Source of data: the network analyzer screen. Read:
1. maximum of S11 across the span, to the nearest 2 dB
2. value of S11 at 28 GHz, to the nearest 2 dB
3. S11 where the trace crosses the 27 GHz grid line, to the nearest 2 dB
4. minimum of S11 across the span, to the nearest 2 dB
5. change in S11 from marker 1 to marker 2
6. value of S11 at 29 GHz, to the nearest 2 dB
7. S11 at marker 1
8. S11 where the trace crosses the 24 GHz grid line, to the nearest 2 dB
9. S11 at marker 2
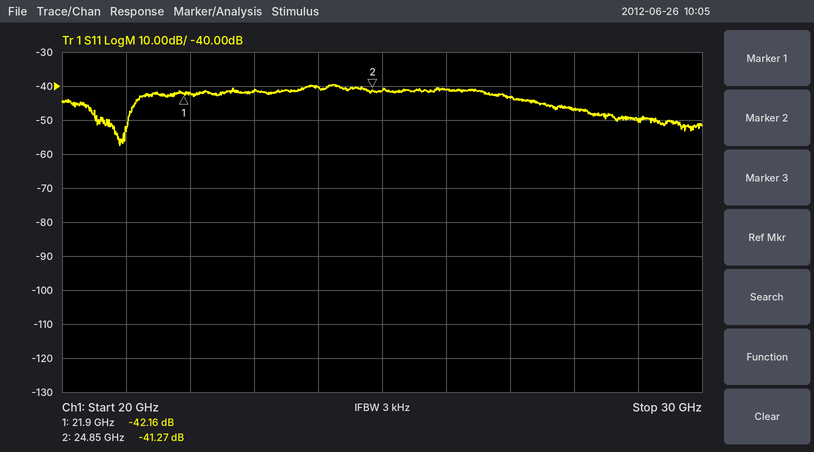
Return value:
-40 dB
-46 dB
-44 dB
-58 dB
0.89 dB
-50 dB
-42.16 dB
-40 dB
-41.27 dB
